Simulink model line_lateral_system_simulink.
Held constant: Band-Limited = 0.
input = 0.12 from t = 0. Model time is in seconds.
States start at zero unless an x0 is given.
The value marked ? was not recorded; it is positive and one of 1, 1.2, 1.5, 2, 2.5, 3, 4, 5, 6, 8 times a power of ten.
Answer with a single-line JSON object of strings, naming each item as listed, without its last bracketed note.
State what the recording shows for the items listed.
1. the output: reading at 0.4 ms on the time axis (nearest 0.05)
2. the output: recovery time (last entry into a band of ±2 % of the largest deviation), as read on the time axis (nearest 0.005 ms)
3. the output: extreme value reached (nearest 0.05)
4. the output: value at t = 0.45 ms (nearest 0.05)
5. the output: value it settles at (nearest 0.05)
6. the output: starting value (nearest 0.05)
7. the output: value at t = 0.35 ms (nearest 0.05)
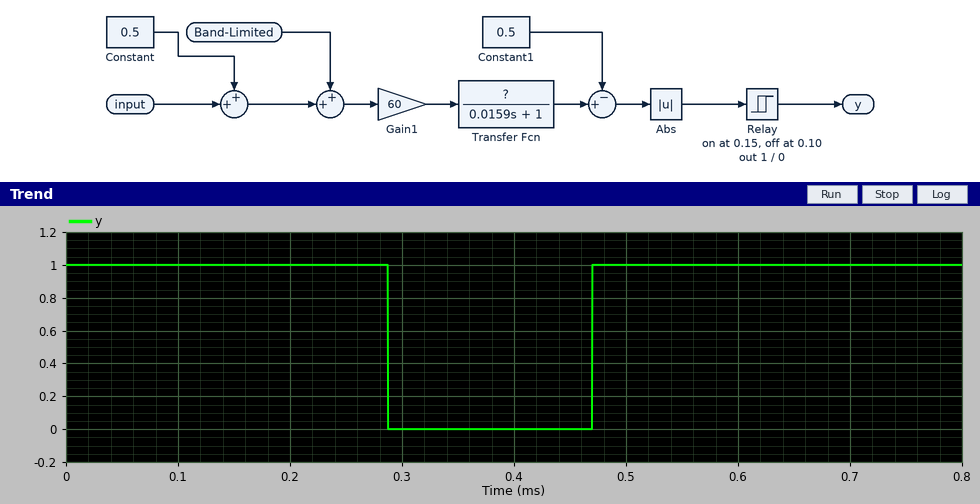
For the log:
{"the output: reading at 0.4 ms on the time axis": "0.00", "the output: recovery time (last entry into a band of ±2 % of the largest deviation), as read on the time axis": "0.470 ms", "the output: extreme value reached": "0.00", "the output: value at t = 0.45 ms": "0.00", "the output: value it settles at": "1.00", "the output: starting value": "1.00", "the output: value at t = 0.35 ms": "0.00"}
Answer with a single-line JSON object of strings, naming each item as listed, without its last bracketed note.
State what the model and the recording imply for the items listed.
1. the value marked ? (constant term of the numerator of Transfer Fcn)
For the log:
{"the value marked ?": "0.6"}
